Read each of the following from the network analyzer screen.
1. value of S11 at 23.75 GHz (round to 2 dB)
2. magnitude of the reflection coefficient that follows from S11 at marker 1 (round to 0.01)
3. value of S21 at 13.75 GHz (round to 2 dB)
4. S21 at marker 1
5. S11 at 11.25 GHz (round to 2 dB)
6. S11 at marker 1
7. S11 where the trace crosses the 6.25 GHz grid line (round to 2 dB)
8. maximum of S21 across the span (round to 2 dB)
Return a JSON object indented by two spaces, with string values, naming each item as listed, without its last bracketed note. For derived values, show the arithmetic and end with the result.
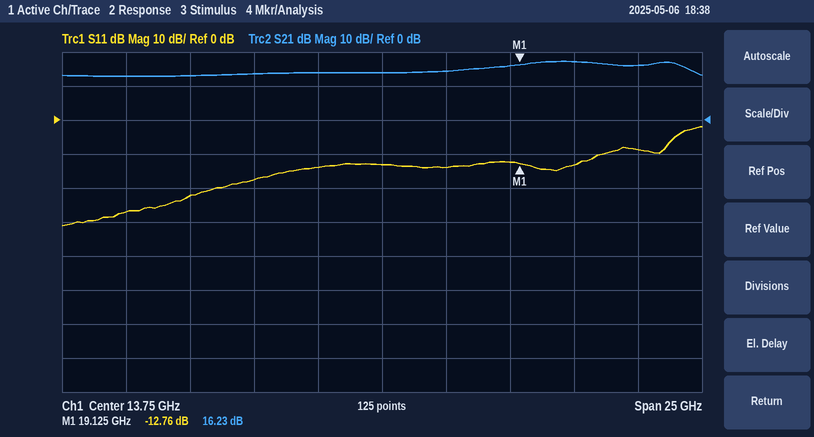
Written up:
{
  "value of S11 at 23.75 GHz": "-8 dB",
  "magnitude of the reflection coefficient that follows from S11 at marker 1": "10^(-12.76/20) ≈ 0.23",
  "value of S21 at 13.75 GHz": "14 dB",
  "S21 at marker 1": "16.23 dB",
  "S11 at 11.25 GHz": "-14 dB",
  "S11 at marker 1": "-12.76 dB",
  "S11 where the trace crosses the 6.25 GHz grid line": "-22 dB",
  "maximum of S21 across the span": "18 dB"
}
